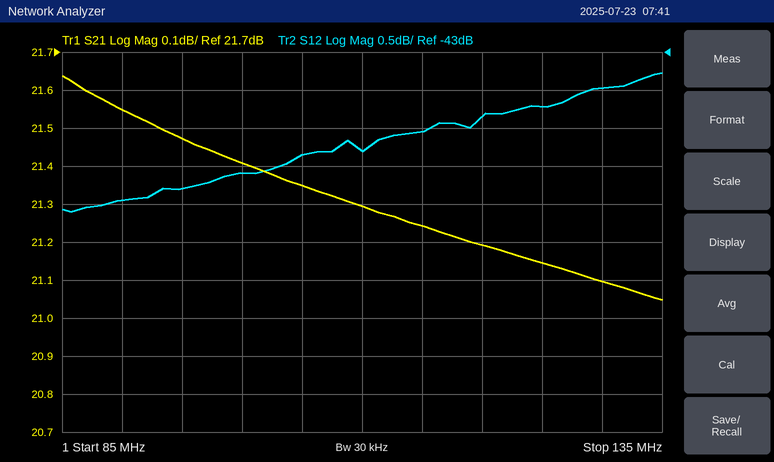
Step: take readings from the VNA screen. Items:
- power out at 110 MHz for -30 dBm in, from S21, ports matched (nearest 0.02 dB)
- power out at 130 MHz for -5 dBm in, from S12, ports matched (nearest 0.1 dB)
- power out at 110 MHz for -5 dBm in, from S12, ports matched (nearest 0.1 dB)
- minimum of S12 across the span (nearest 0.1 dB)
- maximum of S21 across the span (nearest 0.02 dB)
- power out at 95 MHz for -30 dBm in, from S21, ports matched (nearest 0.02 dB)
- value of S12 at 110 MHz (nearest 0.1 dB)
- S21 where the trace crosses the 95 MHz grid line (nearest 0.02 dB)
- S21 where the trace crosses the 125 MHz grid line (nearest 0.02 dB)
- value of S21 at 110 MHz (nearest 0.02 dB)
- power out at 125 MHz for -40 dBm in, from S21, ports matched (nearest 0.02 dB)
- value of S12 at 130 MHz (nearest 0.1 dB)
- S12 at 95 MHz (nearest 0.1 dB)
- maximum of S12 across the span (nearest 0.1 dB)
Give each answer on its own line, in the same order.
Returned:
-8.70 dBm
-48.5 dBm
-49.3 dBm
-45.1 dB
21.64 dB
-8.52 dBm
-44.3 dB
21.48 dB
21.14 dB
21.30 dB
-18.86 dBm
-43.5 dB
-44.8 dB
-43.3 dB
